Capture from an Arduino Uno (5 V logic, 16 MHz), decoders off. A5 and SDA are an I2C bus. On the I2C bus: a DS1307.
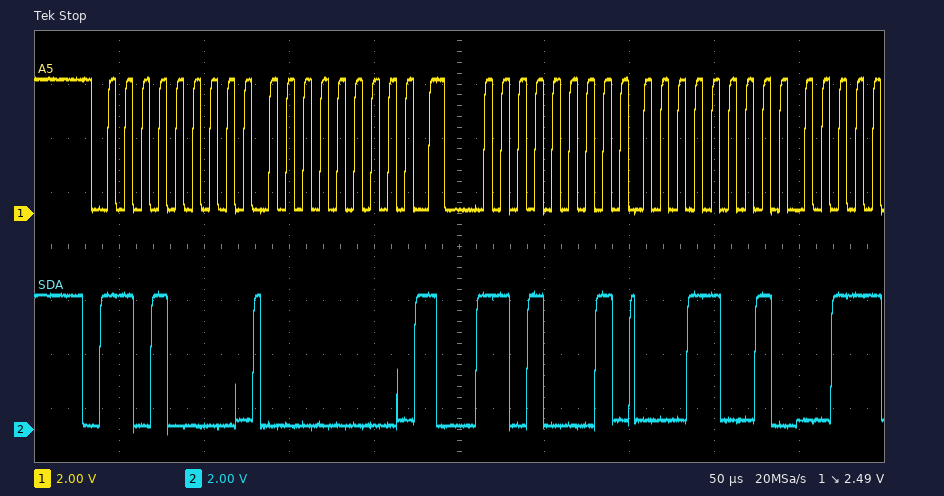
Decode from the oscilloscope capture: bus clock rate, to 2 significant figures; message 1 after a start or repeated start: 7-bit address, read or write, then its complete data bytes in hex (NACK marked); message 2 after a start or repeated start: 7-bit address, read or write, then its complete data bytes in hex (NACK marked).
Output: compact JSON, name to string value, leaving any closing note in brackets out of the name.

{"bus clock rate, to 2 significant figures": "100 kHz", "message 1 after a start or repeated start: 7-bit address, read or write, then its complete data bytes in hex": "0x68 write: 00", "message 2 after a start or repeated start: 7-bit address, read or write, then its complete data bytes in hex": "0x68 read: 19"}
